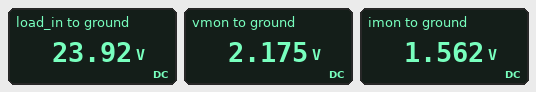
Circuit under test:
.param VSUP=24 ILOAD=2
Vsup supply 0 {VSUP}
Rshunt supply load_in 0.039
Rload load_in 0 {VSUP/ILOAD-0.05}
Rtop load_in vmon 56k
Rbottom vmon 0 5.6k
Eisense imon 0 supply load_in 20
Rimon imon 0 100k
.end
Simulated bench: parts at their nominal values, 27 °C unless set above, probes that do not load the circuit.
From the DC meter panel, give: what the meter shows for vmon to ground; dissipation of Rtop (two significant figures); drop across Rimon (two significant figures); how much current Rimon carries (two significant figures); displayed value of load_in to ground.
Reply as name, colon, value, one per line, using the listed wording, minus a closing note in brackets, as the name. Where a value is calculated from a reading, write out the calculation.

what the meter shows for vmon to ground: 2.175 V
dissipation of Rtop: (23.92 V - 2.175 V)^2 / 56 kΩ = 8.4 mW
drop across Rimon: 1.562 V = 1.6 V
how much current Rimon carries: (1.562 V) / 100 kΩ = 16 µA
displayed value of load_in to ground: 23.92 V
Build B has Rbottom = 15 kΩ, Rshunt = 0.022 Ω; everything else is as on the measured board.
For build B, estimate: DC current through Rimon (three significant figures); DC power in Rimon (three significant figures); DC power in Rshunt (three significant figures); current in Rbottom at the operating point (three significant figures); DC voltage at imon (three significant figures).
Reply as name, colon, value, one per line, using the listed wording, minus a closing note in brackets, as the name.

DC current through Rimon: 8.82 µA
DC power in Rimon: 7.78 µW
DC power in Rshunt: 88.4 mW
current in Rbottom at the operating point: 337 µA
DC voltage at imon: 882 mV
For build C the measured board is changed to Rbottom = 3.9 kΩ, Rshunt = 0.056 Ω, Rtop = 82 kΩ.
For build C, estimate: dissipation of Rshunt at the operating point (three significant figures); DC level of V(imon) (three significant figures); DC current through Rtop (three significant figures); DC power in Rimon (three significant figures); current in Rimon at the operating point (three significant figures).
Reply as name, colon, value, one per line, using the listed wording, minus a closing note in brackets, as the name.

dissipation of Rshunt at the operating point: 224 mW
DC level of V(imon): 2.24 V
DC current through Rtop: 278 µA
DC power in Rimon: 50.1 µW
current in Rimon at the operating point: 22.4 µA
